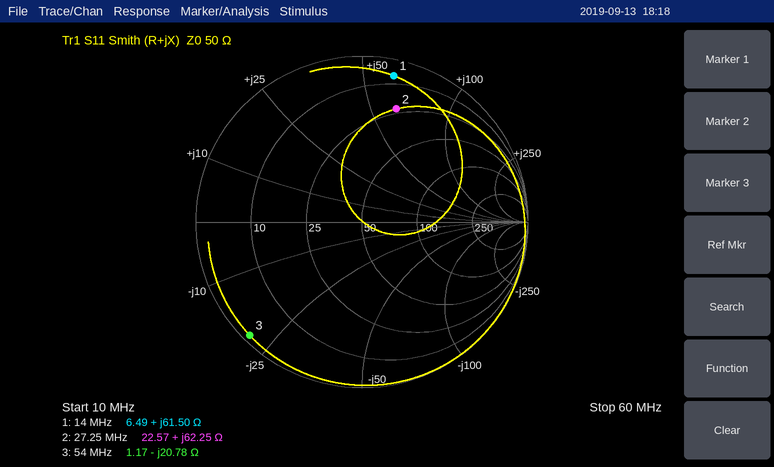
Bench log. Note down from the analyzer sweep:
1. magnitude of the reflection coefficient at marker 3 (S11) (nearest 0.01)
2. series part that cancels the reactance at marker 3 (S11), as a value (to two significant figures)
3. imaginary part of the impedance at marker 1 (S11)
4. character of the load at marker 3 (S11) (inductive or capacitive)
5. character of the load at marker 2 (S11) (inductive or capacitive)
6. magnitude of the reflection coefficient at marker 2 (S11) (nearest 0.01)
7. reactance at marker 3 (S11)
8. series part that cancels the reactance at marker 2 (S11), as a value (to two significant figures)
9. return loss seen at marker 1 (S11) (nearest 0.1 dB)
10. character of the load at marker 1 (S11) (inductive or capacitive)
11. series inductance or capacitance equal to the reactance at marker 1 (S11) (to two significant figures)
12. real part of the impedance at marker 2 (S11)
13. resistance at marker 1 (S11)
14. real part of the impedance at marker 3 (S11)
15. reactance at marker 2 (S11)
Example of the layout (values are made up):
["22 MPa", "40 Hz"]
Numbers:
["0.96", "61 nH", "+61.50 Ω", "capacitive", "inductive", "0.71", "-20.78 Ω", "94 pF", "0.9 dB", "inductive", "700 nH", "22.57 Ω", "6.49 Ω", "1.17 Ω", "+62.25 Ω"]
